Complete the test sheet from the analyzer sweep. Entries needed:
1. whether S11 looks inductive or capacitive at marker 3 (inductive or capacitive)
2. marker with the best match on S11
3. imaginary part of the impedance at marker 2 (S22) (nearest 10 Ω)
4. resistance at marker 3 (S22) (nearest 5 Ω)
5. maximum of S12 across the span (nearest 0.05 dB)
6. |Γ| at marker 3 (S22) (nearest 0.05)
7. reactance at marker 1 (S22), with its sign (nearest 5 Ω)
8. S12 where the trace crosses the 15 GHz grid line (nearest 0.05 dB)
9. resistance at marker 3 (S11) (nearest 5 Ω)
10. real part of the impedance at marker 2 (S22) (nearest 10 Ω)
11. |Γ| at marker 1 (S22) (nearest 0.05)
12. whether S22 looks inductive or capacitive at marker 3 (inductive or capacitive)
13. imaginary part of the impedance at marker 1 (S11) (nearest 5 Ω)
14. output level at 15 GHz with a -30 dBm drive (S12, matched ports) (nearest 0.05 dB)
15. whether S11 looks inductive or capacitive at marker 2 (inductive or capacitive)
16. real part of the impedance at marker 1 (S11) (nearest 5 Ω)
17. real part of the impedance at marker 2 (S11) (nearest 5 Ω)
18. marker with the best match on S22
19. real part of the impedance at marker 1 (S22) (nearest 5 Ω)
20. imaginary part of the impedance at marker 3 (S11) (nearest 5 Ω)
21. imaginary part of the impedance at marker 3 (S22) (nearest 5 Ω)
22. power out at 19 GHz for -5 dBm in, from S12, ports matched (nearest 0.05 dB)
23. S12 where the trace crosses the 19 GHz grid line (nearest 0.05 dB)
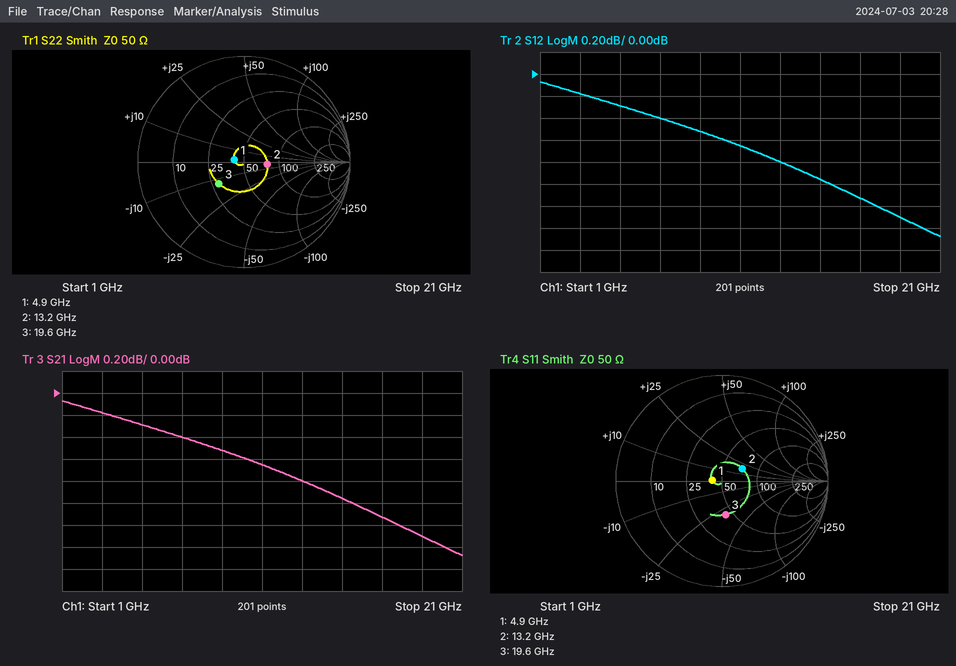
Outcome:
capacitive
marker 1
0 Ω
30 Ω
-0.05 dB
0.30
0 Ω
-0.95 dB
45 Ω
80 Ω
0.10
capacitive
0 Ω
-30.95 dBm
inductive
40 Ω
70 Ω
marker 1
40 Ω
-30 Ω
-15 Ω
-6.30 dBm
-1.30 dB
